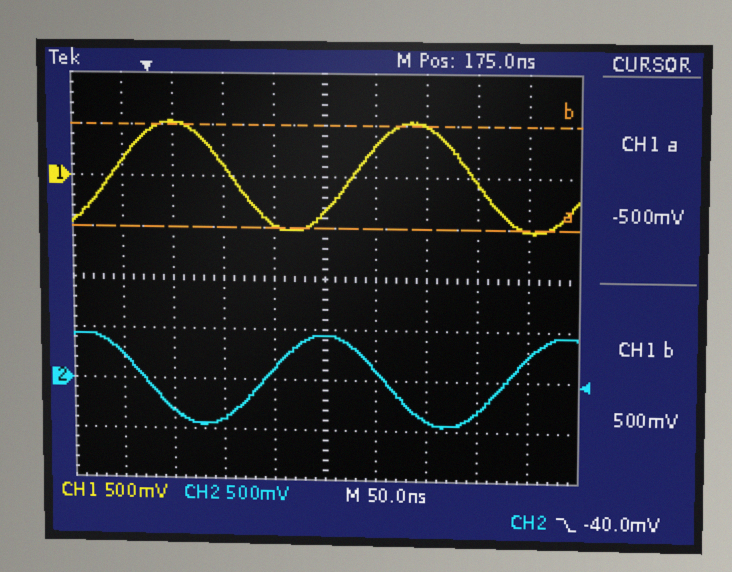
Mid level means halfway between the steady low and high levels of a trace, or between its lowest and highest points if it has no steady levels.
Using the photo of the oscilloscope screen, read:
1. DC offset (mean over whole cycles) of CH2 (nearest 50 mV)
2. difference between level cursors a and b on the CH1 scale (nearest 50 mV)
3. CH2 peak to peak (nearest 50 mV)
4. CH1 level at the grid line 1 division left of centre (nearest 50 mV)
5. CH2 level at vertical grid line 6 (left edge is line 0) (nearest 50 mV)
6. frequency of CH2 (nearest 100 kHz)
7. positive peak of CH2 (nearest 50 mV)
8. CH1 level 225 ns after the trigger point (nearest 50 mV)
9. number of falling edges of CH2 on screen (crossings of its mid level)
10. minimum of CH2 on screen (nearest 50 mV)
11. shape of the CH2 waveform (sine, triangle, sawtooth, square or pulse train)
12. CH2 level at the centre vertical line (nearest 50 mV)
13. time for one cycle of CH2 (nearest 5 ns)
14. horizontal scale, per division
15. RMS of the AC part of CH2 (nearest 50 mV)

0 mV
1.00 V
900 mV
-450 mV
100 mV
4.2 MHz
450 mV
300 mV
2
-450 mV
sine
450 mV
240 ns
50 ns
300 mV
